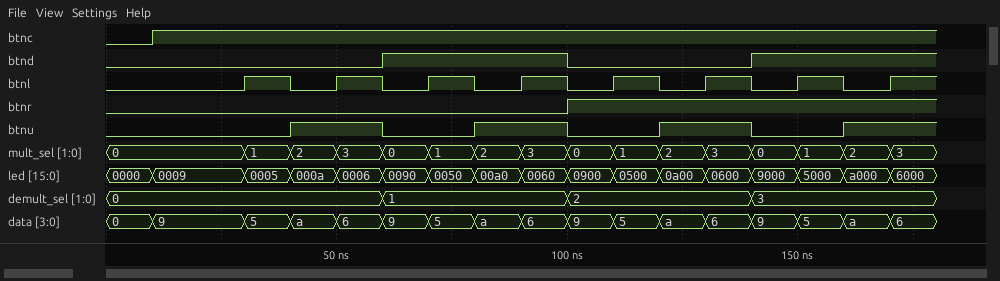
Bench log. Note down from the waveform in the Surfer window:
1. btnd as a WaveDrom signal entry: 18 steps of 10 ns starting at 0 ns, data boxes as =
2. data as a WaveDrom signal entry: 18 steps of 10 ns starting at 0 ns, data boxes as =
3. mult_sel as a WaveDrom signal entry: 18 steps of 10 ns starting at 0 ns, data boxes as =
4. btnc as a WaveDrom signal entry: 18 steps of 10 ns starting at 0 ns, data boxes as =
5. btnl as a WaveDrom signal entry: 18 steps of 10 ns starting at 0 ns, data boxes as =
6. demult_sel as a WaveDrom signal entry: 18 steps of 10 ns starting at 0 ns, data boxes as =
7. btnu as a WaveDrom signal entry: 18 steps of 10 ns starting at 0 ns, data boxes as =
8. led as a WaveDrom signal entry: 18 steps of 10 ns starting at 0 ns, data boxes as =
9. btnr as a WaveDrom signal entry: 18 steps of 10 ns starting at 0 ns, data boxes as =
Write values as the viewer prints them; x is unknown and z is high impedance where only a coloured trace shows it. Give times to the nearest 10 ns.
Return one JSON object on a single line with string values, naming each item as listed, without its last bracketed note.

{"btnd as a WaveDrom signal entry: 18 steps of 10 ns starting at 0 ns, data boxes as =": "{name: 'btnd', wave: '0.....1...0...1...'}", "data as a WaveDrom signal entry: 18 steps of 10 ns starting at 0 ns, data boxes as =": "{name: 'data', wave: '==.===============', data: '0 9 5 a 6 9 5 a 6 9 5 a 6 9 5 a 6'}", "mult_sel as a WaveDrom signal entry: 18 steps of 10 ns starting at 0 ns, data boxes as =": "{name: 'mult_sel', wave: '=..===============', data: '0 1 2 3 0 1 2 3 0 1 2 3 0 1 2 3'}", "btnc as a WaveDrom signal entry: 18 steps of 10 ns starting at 0 ns, data boxes as =": "{name: 'btnc', wave: '01................'}", "btnl as a WaveDrom signal entry: 18 steps of 10 ns starting at 0 ns, data boxes as =": "{name: 'btnl', wave: '0..101010101010101'}", "demult_sel as a WaveDrom signal entry: 18 steps of 10 ns starting at 0 ns, data boxes as =": "{name: 'demult_sel', wave: '=.....=...=...=...', data: '0 1 2 3'}", "btnu as a WaveDrom signal entry: 18 steps of 10 ns starting at 0 ns, data boxes as =": "{name: 'btnu', wave: '0...1.0.1.0.1.0.1.'}", "led as a WaveDrom signal entry: 18 steps of 10 ns starting at 0 ns, data boxes as =": "{name: 'led', wave: '==.===============', data: '0000 0009 0005 000a 0006 0090 0050 00a0 0060 0900 0500 0a00 0600 9000 5000 a000 6000'}", "btnr as a WaveDrom signal entry: 18 steps of 10 ns starting at 0 ns, data boxes as =": "{name: 'btnr', wave: '0.........1.......'}"}
